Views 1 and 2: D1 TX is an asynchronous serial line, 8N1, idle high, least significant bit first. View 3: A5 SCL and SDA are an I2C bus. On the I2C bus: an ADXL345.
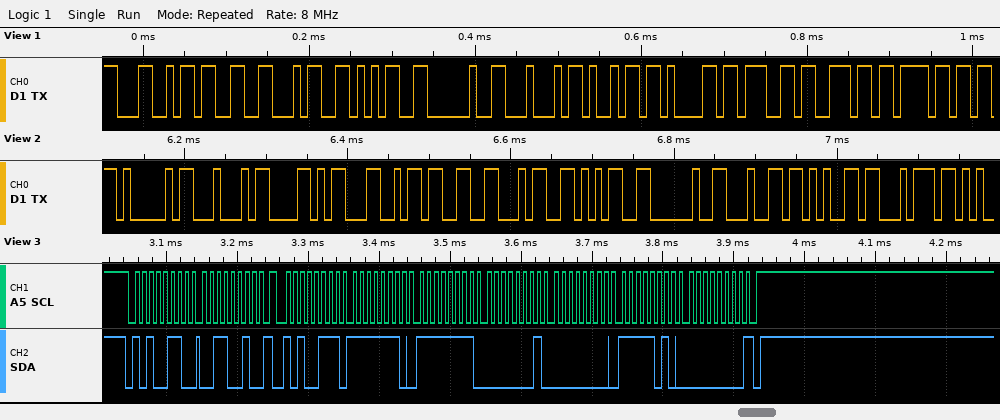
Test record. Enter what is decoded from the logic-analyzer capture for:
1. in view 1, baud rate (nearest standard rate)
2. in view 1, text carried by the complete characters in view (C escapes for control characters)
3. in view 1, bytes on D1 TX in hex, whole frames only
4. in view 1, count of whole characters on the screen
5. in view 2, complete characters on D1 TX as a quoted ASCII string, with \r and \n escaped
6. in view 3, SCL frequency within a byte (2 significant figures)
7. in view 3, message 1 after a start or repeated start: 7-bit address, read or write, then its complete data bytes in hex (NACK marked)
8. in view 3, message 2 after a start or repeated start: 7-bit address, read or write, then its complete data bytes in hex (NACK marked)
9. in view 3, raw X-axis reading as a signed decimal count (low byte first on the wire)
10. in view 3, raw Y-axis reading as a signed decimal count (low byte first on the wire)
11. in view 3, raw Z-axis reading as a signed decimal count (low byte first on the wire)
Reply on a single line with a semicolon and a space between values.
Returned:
115200 baud; "L345 Diagno"; 0x4C 0x33 0x34 0x35 0x20 0x44 0x69 0x61 0x67 0x6E 0x6F; 11; "ADXL345 det"; 100 kHz; 0x53 write: 32; 0x53 read: FE FF 01 00 FA 00 NACK; -2; 1; 250
